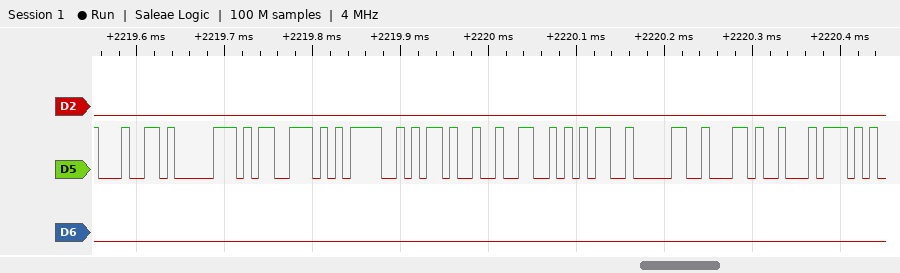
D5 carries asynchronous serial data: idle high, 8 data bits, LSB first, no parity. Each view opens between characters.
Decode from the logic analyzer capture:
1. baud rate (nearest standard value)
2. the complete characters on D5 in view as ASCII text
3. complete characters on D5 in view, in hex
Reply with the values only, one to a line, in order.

115200 baud
"dps=-250,t"
64, 70, 73, 3D, 2D, 32, 35, 30, 2C, 74
